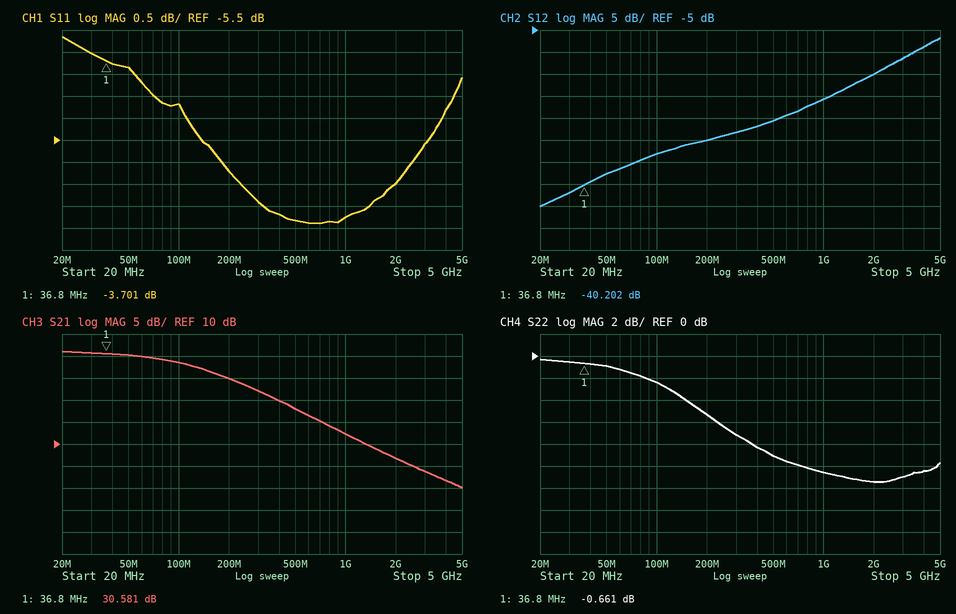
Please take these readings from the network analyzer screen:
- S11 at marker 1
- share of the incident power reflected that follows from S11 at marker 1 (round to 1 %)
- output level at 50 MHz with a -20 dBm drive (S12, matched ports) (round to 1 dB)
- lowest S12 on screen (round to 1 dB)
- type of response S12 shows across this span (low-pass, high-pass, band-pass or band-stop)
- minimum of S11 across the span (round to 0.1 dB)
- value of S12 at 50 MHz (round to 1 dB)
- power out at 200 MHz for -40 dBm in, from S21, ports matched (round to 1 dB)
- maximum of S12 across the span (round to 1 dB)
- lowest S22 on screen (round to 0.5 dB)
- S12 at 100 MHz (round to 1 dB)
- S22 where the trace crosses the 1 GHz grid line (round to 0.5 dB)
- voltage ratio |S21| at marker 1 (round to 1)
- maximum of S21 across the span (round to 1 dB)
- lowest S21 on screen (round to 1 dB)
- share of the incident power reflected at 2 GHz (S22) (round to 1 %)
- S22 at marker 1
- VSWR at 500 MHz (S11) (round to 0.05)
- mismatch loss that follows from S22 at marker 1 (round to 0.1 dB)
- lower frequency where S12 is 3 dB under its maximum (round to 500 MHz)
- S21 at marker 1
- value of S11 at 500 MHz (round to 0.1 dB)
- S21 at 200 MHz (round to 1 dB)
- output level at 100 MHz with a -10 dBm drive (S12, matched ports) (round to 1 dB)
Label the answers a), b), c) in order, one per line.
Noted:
a) -3.701 dB
b) 43 %
c) -58 dBm
d) -45 dB
e) high-pass
f) -7.4 dB
g) -38 dB
h) -15 dBm
i) -7 dB
j) -11.5 dB
k) -33 dB
l) -10.5 dB
m) 34
n) 31 dB
o) 0 dB
p) 7 %
q) -0.661 dB
r) 2.50
s) 8.5 dB
t) 3.5 GHz
u) 30.581 dB
v) -7.3 dB
w) 25 dB
x) -43 dBm
